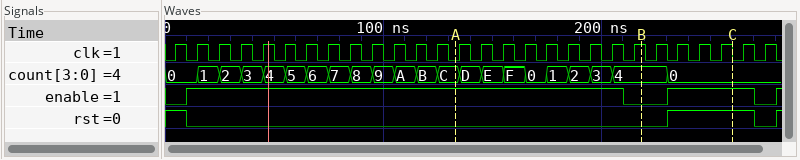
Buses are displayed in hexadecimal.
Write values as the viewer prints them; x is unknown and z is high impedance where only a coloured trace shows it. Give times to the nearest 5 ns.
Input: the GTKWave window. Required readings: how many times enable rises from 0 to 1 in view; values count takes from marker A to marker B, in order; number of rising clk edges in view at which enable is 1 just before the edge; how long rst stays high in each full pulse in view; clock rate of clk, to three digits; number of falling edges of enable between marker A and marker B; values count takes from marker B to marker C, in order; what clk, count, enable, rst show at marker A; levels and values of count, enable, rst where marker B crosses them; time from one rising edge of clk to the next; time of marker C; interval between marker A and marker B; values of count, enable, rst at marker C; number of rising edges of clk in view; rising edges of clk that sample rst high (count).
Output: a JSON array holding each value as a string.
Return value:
["3", "C, D, E, F, 0, 1, 2, 3, 4", "24", "40 ns", "100 MHz", "1", "4, 0", "clk=0, count=C, enable=1, rst=0", "count=4, enable=0, rst=0", "10 ns", "260 ns", "85 ns", "count=0, enable=1, rst=1", "28", "5"]
